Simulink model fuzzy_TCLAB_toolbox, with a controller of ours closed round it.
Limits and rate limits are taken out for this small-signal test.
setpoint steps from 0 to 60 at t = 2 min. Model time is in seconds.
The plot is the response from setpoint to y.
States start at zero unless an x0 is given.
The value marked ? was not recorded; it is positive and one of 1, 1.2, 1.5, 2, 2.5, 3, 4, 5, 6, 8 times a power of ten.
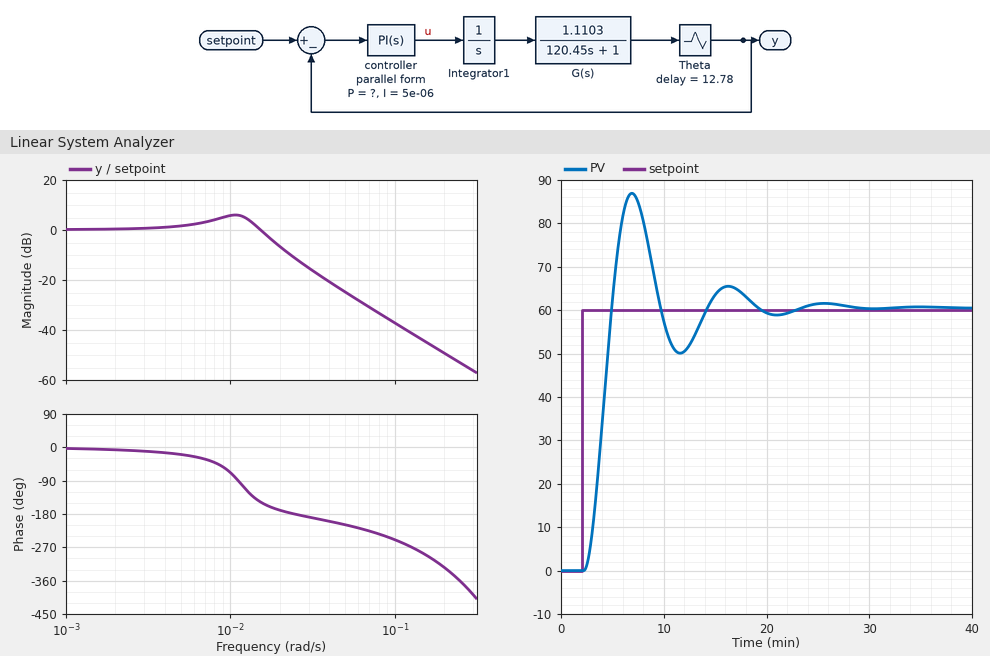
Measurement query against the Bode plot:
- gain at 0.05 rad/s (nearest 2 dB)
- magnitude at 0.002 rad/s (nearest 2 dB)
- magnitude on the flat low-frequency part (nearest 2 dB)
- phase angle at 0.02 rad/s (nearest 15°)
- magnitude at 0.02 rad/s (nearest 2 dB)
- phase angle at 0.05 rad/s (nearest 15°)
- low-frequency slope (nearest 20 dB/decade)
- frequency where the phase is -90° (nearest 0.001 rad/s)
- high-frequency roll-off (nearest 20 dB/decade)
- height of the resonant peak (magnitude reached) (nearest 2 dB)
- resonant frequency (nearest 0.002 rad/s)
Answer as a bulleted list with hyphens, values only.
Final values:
- -24 dB
- 0 dB
- 0 dB
- -165°
- -6 dB
- -210°
- 0 dB/decade
- 0.011 rad/s
- -40 dB/decade
- 6 dB
- 0.010 rad/s
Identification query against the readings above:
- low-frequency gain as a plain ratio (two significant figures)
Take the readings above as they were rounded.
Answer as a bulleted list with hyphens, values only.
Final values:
- 1.0
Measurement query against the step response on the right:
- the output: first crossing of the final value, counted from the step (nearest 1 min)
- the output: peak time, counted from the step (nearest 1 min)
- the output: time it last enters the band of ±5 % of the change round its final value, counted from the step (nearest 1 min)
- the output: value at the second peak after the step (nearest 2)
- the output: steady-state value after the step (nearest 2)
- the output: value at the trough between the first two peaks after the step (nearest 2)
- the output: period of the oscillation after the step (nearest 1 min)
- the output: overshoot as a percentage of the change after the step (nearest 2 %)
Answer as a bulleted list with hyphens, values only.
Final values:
- 3 min
- 5 min
- 16 min
- 66
- 60
- 50
- 9 min
- 44 %
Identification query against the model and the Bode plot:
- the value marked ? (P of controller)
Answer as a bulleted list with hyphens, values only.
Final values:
- 0.015
